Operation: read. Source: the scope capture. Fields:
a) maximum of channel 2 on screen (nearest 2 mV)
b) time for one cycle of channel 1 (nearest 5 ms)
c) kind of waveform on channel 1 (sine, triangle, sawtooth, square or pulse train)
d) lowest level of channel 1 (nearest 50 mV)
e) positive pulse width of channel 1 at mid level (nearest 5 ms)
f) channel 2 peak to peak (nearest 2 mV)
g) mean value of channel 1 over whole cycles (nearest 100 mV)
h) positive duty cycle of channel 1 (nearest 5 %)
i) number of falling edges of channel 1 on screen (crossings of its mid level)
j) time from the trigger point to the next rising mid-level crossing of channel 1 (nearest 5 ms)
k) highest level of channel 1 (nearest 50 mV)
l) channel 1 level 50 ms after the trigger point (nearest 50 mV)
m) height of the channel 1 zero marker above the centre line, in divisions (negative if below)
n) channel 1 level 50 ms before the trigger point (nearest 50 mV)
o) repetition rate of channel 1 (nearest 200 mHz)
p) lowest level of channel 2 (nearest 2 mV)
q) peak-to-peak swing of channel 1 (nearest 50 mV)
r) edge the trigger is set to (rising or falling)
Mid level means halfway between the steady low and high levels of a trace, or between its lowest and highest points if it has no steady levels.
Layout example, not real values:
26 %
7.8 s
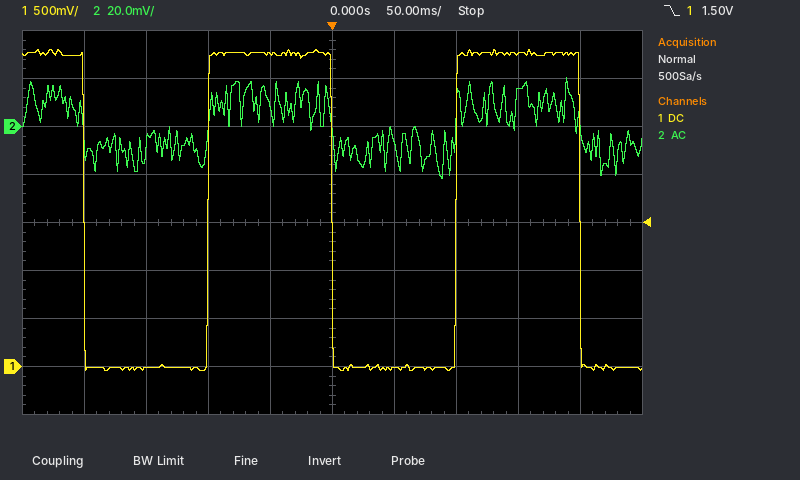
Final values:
20 mV
200 ms
square
-50 mV
100 ms
42 mV
1.6 V
50 %
3
100 ms
3.30 V
0 mV
-3.0 div
3.25 V
5.0 Hz
-22 mV
3.35 V
falling
